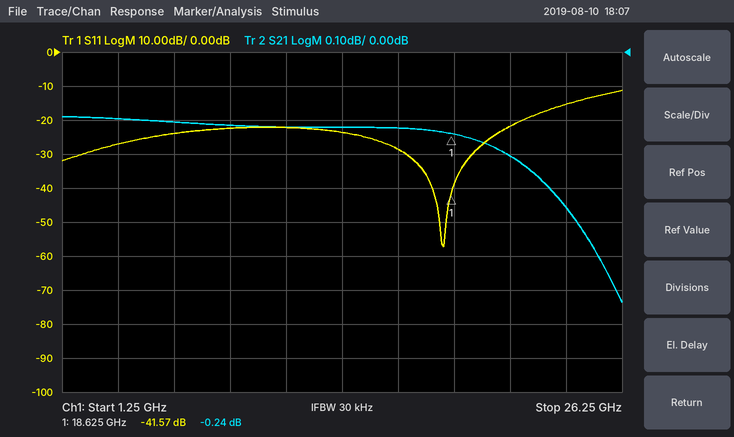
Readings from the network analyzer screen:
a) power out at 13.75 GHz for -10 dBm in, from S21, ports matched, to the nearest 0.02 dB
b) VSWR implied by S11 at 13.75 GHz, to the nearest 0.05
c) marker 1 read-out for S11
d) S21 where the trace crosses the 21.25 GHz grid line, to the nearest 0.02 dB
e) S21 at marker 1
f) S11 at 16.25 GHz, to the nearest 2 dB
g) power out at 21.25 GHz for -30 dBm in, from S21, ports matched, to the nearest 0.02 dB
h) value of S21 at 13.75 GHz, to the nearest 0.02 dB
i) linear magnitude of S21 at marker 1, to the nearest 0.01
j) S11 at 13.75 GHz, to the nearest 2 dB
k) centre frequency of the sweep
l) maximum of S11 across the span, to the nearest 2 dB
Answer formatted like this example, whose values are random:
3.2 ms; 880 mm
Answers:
-10.22 dBm; 1.15; -41.57 dB; -0.30 dB; -0.24 dB; -28 dB; -30.30 dBm; -0.22 dB; 0.97; -24 dB; 13.75 GHz; -12 dB
